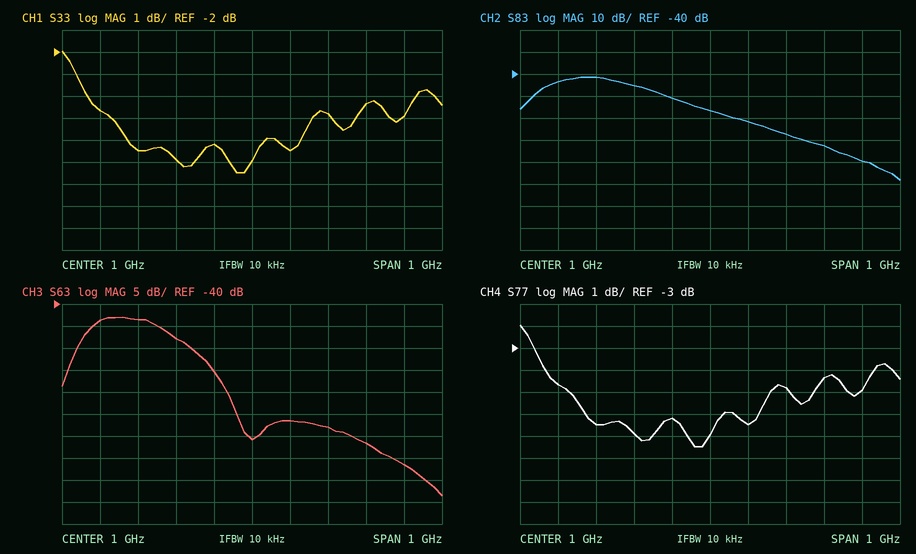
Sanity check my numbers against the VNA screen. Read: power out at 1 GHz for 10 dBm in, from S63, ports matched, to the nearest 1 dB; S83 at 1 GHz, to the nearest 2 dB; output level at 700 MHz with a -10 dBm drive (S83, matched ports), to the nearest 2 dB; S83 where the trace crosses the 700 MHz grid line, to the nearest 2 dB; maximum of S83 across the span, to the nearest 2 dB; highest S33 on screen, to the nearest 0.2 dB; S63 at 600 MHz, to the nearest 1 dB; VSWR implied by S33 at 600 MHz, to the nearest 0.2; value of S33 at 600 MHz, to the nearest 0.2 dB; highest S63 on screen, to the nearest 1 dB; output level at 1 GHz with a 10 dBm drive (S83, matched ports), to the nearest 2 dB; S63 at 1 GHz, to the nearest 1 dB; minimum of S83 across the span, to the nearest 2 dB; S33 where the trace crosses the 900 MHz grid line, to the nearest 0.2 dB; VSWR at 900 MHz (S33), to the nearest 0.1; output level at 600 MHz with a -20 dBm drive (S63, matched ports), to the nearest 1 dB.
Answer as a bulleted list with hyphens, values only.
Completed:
- -61 dBm
- -56 dB
- -52 dBm
- -42 dB
- -42 dB
- -2.0 dB
- -44 dB
- 3.8
- -4.6 dB
- -43 dB
- -46 dBm
- -71 dB
- -88 dB
- -6.2 dB
- 2.9
- -64 dBm
